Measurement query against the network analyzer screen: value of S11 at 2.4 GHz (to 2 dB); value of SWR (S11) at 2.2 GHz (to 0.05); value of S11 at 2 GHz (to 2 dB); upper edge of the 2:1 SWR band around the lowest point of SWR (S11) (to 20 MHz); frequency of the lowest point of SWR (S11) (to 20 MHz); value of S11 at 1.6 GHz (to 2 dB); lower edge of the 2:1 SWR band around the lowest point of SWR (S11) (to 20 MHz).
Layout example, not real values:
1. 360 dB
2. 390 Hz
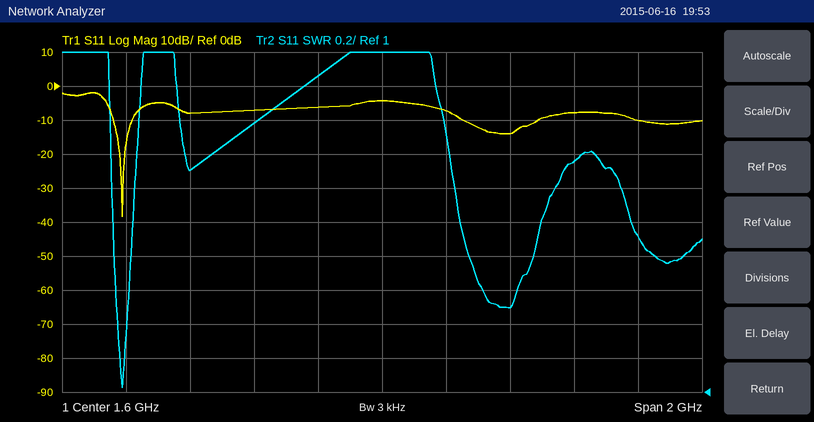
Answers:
1. -10 dB
2. 2.35
3. -14 dB
4. 820 MHz
5. 780 MHz
6. -4 dB
7. 760 MHz
